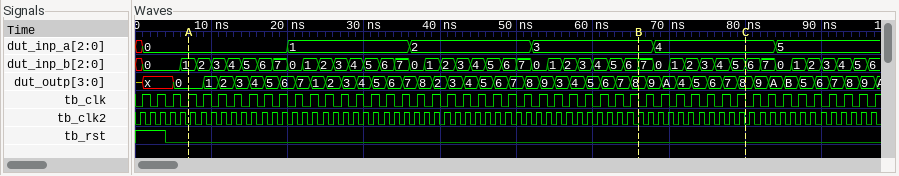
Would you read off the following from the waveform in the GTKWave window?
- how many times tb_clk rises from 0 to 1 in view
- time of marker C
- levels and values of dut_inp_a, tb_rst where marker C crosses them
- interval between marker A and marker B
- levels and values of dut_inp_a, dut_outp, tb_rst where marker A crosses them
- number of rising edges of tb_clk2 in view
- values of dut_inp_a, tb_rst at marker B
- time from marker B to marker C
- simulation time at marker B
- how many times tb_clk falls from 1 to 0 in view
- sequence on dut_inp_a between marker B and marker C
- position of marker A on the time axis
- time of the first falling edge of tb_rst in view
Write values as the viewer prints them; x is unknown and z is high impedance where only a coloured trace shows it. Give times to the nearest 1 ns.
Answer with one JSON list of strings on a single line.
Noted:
["49", "80 ns", "dut_inp_a=4, tb_rst=0", "59 ns", "dut_inp_a=0, dut_outp=0, tb_rst=0", "73", "dut_inp_a=3, tb_rst=0", "14 ns", "66 ns", "48", "3, 4", "7 ns", "4 ns"]
